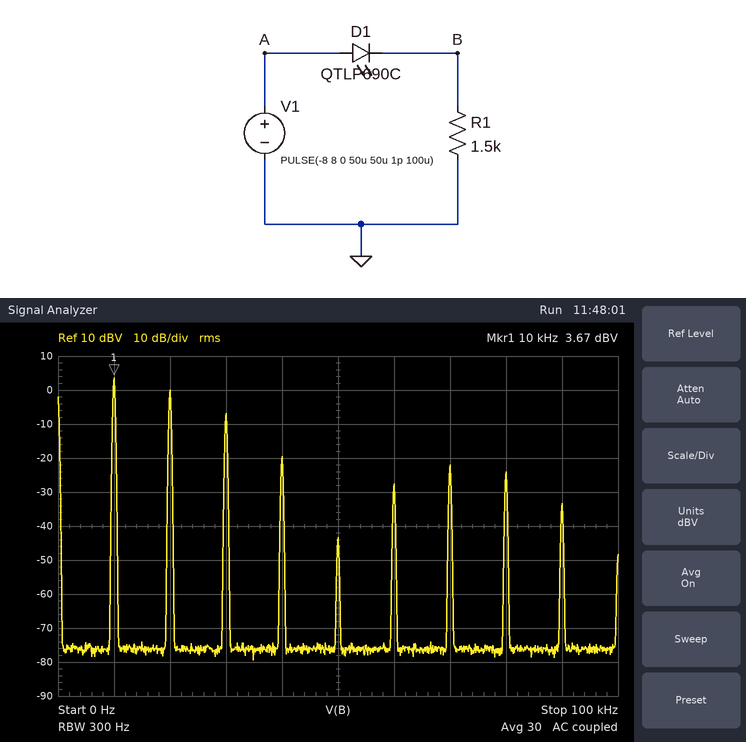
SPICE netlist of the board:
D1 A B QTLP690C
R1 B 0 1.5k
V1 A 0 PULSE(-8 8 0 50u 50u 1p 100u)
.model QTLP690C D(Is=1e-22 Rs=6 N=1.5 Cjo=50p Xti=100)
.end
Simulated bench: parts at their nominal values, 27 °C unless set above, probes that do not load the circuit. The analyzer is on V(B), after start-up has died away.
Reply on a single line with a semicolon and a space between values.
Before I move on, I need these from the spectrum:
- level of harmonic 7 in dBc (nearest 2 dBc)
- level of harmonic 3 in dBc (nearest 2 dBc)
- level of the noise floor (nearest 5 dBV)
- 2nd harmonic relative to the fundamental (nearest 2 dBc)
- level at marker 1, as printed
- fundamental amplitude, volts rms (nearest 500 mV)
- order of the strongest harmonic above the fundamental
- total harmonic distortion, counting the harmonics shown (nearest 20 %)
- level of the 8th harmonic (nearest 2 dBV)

-26 dBc; -10 dBc; -75 dBV; -4 dBc; 3.67 dBV; 1.5 V; 2; 80 %; -24 dBV
